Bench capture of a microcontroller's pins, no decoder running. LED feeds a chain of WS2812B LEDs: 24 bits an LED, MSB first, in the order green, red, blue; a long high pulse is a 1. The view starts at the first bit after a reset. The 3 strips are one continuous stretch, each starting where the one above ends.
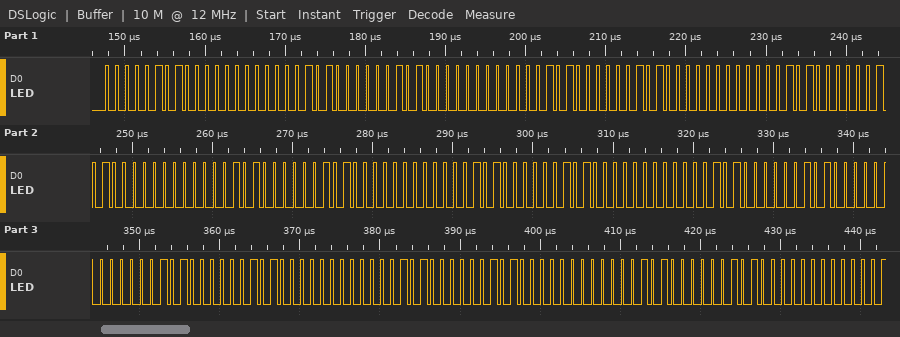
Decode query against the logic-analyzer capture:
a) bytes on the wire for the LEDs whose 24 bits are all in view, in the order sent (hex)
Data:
05 00 0A 05 00 0A 05 00 0A 05 00 0A 05 00 0A 05 00 0A 05 00 0A 05 00 0A 05 00 0A
